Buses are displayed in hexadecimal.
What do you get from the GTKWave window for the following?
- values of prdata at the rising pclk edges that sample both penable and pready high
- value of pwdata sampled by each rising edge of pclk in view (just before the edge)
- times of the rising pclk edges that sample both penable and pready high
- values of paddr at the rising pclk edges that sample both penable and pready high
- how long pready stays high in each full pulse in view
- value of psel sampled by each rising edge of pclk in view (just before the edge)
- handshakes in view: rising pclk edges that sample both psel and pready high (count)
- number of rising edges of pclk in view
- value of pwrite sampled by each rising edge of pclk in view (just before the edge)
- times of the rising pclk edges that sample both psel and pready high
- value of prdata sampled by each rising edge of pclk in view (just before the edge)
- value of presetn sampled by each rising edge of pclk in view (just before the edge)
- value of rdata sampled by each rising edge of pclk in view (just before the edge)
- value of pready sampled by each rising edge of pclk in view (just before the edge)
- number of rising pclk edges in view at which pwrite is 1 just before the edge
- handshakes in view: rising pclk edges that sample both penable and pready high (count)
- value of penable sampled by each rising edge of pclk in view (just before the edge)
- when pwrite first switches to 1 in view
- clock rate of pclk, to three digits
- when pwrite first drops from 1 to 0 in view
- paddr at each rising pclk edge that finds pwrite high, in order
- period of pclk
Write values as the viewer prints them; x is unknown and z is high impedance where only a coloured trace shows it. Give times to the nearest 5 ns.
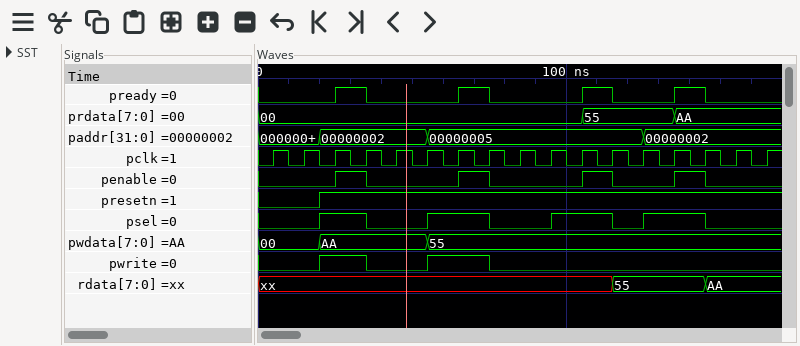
00, 00, 55, AA
00, 00, AA, AA, AA, AA, 55, 55, 55, 55, 55, 55, 55, 55, 55, 55, 55
35 ns, 75 ns, 115 ns, 145 ns
00000002, 00000005, 00000005, 00000002
10 ns, 10 ns, 10 ns, 10 ns
0 0 1 1 0 0 1 1 0 0 1 1 0 1 1 0 0
4
17
0 0 1 1 0 0 1 1 0 0 0 0 0 0 0 0 0
35 ns, 75 ns, 115 ns, 145 ns
00, 00, 00, 00, 00, 00, 00, 00, 00, 00, 00, 55, 55, 55, AA, AA, AA
0 0 1 1 1 1 1 1 1 1 1 1 1 1 1 1 1
xx, xx, xx, xx, xx, xx, xx, xx, xx, xx, xx, xx, 55, 55, 55, AA, AA
0 0 0 1 0 0 0 1 0 0 0 1 0 0 1 0 0
4
4
0 0 0 1 0 0 0 1 0 0 0 1 0 0 1 0 0
20 ns
100 MHz
35 ns
00000002, 00000002, 00000005, 00000005
10 ns
